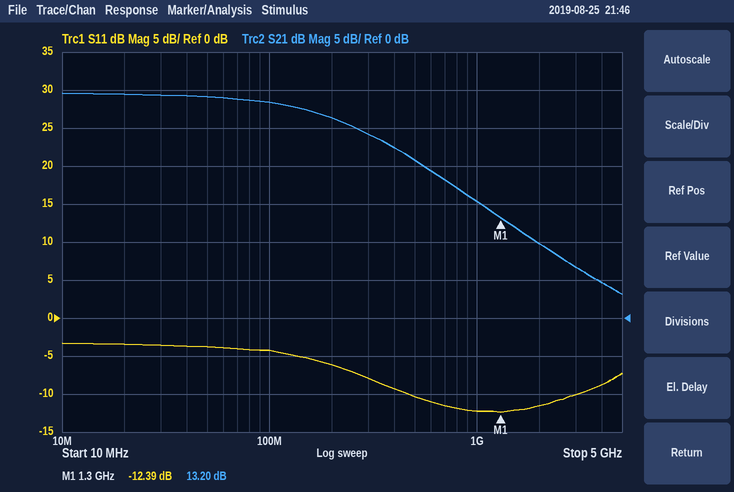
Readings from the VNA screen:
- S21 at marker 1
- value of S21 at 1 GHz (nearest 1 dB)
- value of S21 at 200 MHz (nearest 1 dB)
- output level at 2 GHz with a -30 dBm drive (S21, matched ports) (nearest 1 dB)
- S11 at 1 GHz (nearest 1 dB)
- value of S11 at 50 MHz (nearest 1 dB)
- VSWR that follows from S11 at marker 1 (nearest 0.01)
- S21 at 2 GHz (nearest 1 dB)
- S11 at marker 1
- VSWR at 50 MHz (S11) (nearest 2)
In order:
13.20 dB
15 dB
26 dB
-20 dBm
-12 dB
-4 dB
1.63
10 dB
-12.39 dB
4
